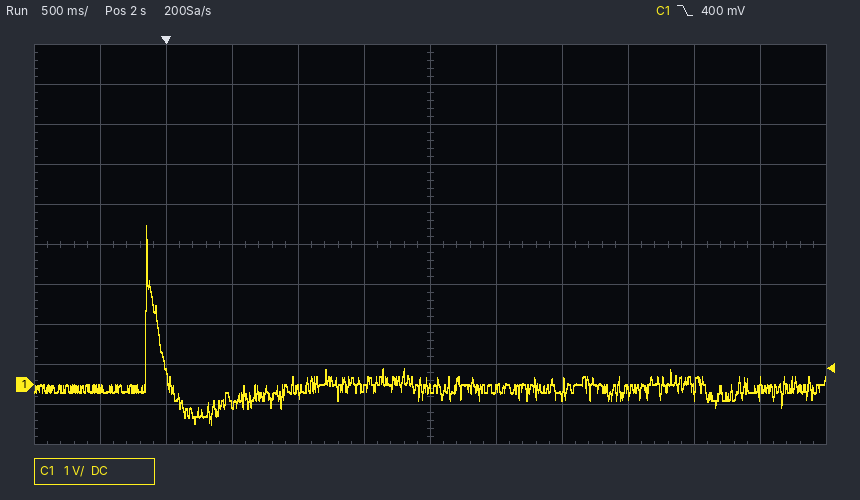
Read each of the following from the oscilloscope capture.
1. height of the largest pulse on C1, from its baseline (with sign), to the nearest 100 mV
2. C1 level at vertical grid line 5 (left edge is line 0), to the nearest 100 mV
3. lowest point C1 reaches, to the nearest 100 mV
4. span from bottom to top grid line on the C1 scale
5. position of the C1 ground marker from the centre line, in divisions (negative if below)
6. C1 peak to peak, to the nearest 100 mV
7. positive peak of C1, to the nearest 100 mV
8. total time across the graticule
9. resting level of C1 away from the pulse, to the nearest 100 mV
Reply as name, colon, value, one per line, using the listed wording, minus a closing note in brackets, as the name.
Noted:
height of the largest pulse on C1, from its baseline (with sign), to the nearest 100 mV: +4.1 V
C1 level at vertical grid line 5 (left edge is line 0), to the nearest 100 mV: -100 mV
lowest point C1 reaches, to the nearest 100 mV: -1.0 V
span from bottom to top grid line on the C1 scale: 10 V
position of the C1 ground marker from the centre line, in divisions: -3.5 div
C1 peak to peak, to the nearest 100 mV: 5.0 V
positive peak of C1, to the nearest 100 mV: 4.0 V
total time across the graticule: 6 s
resting level of C1 away from the pulse, to the nearest 100 mV: -100 mV
